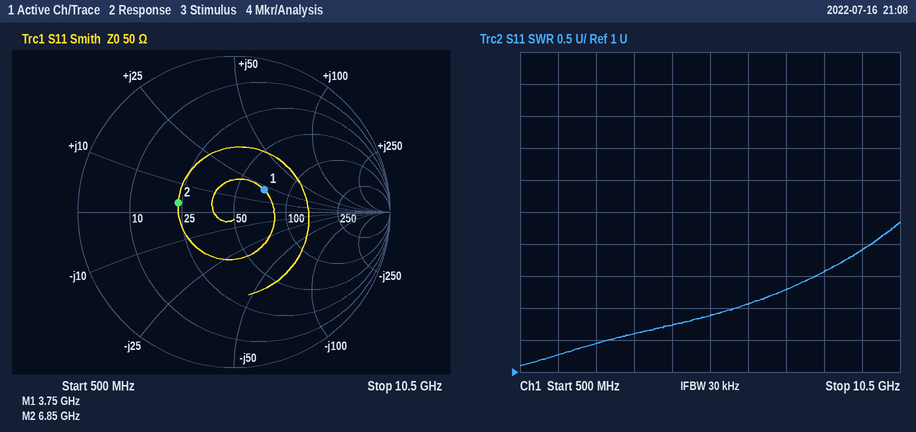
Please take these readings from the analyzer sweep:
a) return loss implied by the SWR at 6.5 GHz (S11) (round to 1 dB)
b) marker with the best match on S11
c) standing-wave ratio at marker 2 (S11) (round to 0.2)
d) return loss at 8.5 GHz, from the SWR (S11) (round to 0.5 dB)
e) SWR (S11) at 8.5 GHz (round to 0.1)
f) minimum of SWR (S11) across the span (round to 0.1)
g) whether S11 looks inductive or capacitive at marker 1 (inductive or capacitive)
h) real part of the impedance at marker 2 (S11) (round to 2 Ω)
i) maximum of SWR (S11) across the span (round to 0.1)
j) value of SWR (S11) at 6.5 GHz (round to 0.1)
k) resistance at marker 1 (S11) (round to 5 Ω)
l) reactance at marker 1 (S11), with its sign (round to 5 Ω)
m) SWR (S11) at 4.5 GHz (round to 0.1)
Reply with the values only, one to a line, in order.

9 dB
marker 1
2.2
7.0 dB
2.6
1.1
inductive
24 Ω
3.3
2.1
70 Ω
+20 Ω
1.7
